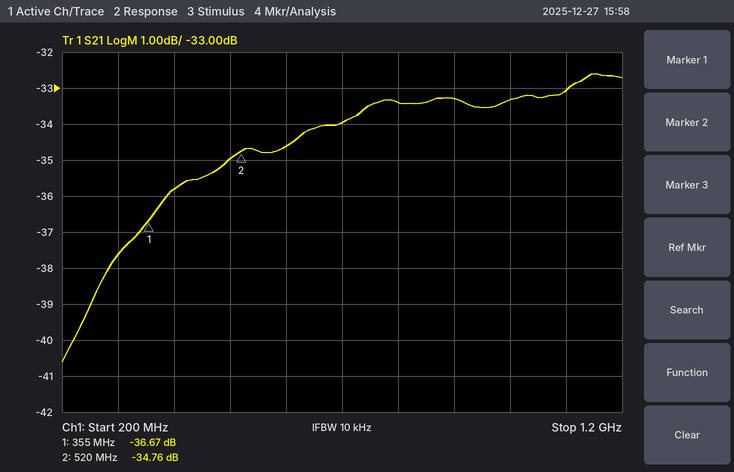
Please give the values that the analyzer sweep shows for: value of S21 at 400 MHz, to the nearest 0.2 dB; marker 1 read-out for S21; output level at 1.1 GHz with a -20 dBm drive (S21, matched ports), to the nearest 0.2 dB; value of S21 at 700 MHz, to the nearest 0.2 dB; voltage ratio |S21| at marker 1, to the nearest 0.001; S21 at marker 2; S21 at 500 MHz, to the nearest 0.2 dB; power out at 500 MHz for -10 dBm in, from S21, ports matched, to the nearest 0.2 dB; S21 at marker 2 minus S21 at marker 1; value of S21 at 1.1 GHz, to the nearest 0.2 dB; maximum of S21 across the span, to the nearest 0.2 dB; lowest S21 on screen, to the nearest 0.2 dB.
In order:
-35.8 dB
-36.67 dB
-53.0 dBm
-34.0 dB
0.015
-34.76 dB
-35.0 dB
-45.0 dBm
1.91 dB
-33.0 dB
-32.6 dB
-40.6 dB
